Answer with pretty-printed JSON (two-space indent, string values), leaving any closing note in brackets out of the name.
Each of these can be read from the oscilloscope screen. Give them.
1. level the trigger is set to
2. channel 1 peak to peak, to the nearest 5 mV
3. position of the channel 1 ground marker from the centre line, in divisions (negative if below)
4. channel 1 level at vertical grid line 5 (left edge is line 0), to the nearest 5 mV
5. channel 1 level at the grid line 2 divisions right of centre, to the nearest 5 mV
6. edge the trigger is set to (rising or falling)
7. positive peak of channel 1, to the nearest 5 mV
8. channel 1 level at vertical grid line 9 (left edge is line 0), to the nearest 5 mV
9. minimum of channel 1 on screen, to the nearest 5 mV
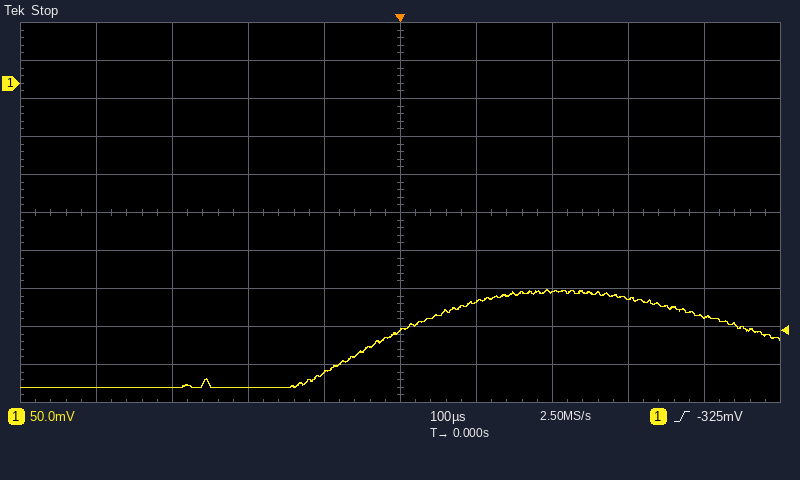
{
  "level the trigger is set to": "-325 mV",
  "channel 1 peak to peak, to the nearest 5 mV": "130 mV",
  "position of the channel 1 ground marker from the centre line, in divisions": "+3.4 div",
  "channel 1 level at vertical grid line 5 (left edge is line 0), to the nearest 5 mV": "-325 mV",
  "channel 1 level at the grid line 2 divisions right of centre, to the nearest 5 mV": "-275 mV",
  "edge the trigger is set to": "rising",
  "positive peak of channel 1, to the nearest 5 mV": "-270 mV",
  "channel 1 level at vertical grid line 9 (left edge is line 0), to the nearest 5 mV": "-305 mV",
  "minimum of channel 1 on screen, to the nearest 5 mV": "-400 mV"
}
